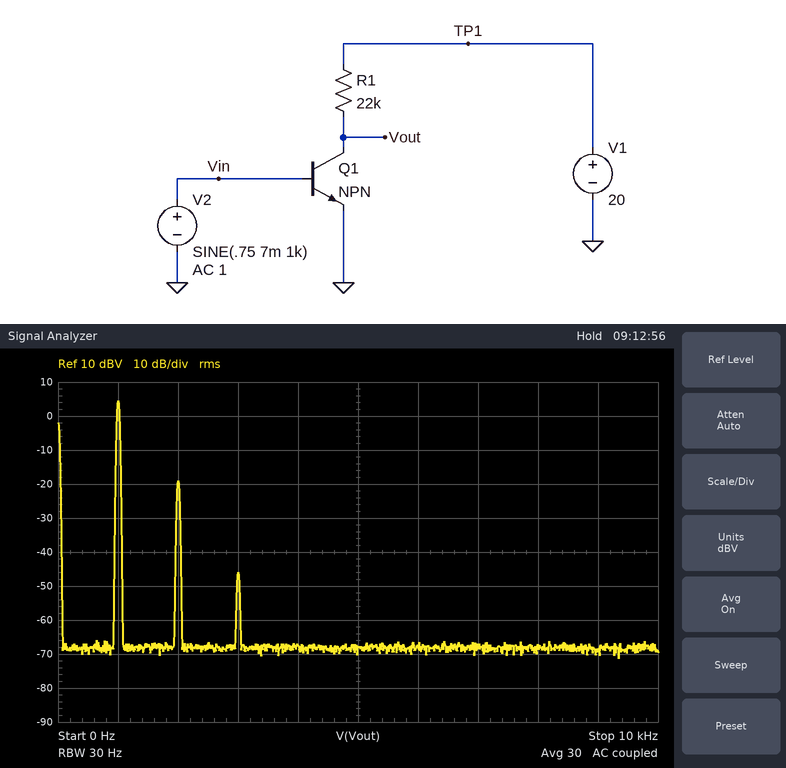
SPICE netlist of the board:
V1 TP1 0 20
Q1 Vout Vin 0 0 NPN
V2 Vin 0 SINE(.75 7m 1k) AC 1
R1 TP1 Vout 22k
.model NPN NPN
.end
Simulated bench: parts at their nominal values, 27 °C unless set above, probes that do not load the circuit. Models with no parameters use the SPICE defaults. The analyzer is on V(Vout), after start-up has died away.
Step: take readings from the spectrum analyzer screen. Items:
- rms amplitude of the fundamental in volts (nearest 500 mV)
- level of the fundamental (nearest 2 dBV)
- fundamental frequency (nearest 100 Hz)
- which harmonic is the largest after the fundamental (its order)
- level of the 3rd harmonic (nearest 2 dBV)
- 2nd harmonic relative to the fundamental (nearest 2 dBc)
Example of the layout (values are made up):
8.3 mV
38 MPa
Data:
1.5 V
4 dBV
1.0 kHz
2
-46 dBV
-24 dBc
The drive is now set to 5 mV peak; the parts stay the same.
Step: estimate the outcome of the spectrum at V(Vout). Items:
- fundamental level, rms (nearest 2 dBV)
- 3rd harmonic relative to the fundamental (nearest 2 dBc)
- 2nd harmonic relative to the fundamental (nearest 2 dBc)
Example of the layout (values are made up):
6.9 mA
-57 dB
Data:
2 dBV
-56 dBc
-26 dBc
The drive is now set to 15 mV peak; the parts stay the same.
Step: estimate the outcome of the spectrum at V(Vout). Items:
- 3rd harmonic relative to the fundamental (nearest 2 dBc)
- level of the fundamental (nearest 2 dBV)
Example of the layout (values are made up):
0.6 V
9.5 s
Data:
-38 dBc
12 dBV
